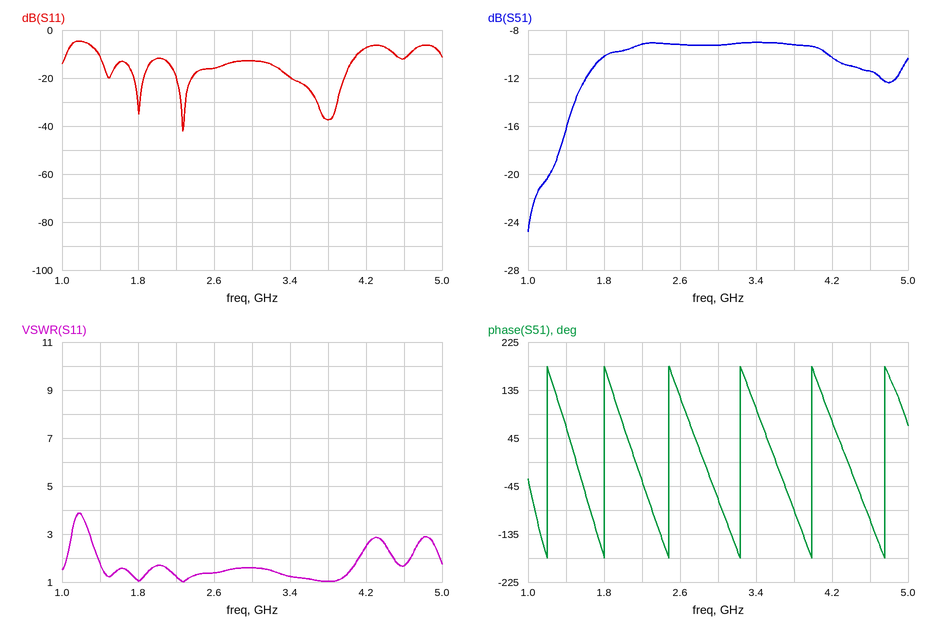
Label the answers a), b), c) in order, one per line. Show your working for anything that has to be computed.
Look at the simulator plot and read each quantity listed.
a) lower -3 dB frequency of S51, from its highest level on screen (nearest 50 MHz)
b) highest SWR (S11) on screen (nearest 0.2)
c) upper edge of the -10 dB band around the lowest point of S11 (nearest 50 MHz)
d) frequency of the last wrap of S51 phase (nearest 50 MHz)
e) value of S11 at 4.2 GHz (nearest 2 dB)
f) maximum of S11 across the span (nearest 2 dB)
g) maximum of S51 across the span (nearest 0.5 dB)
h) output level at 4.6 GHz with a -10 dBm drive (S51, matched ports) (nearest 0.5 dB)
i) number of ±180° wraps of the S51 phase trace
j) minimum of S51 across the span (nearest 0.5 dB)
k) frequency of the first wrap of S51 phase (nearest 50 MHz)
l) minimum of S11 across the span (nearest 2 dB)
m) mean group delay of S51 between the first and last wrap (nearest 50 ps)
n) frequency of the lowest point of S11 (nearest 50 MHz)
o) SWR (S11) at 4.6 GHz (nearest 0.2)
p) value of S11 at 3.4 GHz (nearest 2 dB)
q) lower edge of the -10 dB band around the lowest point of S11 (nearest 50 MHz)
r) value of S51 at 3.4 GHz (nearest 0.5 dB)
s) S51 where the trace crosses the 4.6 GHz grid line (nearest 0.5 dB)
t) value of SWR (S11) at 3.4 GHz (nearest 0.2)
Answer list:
a) 1.60 GHz
b) 3.8
c) 4.10 GHz
d) 4.75 GHz
e) -8 dB
f) -4 dB
g) -9.0 dB
h) -10 dBm + (-11.5 dB) = -21.5 dBm
i) 6
j) -25.0 dB
k) 1.20 GHz
l) -42 dB
m) 5 cycles / (4.75 GHz − 1.20 GHz) ≈ 1.41 ns, so 1.40 ns to the nearest 50 ps
n) 2.25 GHz
o) 1.6
p) -20 dB
q) 1.40 GHz
r) -9.0 dB
s) -11.5 dB
t) 1.2
